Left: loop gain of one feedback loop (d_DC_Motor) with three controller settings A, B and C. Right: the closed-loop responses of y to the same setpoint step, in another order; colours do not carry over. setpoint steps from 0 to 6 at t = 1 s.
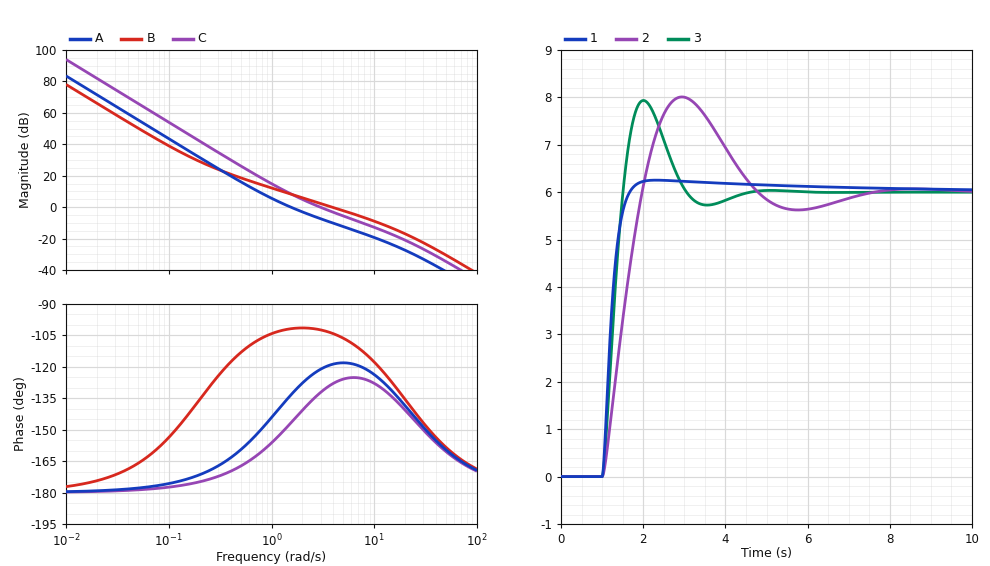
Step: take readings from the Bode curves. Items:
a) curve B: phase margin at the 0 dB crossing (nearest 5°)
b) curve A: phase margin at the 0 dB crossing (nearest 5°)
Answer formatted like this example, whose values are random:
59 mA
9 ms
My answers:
75°
45°
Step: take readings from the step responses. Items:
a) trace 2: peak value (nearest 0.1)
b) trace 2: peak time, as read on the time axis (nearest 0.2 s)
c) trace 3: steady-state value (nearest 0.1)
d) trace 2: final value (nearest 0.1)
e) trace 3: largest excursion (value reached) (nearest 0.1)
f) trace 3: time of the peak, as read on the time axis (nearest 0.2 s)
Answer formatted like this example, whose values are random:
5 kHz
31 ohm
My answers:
8.0
3.0 s
6.0
6.0
7.9
2.0 s
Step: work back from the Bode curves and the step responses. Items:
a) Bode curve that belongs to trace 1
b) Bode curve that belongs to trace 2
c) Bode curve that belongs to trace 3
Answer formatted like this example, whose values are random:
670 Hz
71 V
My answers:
B
A
C
